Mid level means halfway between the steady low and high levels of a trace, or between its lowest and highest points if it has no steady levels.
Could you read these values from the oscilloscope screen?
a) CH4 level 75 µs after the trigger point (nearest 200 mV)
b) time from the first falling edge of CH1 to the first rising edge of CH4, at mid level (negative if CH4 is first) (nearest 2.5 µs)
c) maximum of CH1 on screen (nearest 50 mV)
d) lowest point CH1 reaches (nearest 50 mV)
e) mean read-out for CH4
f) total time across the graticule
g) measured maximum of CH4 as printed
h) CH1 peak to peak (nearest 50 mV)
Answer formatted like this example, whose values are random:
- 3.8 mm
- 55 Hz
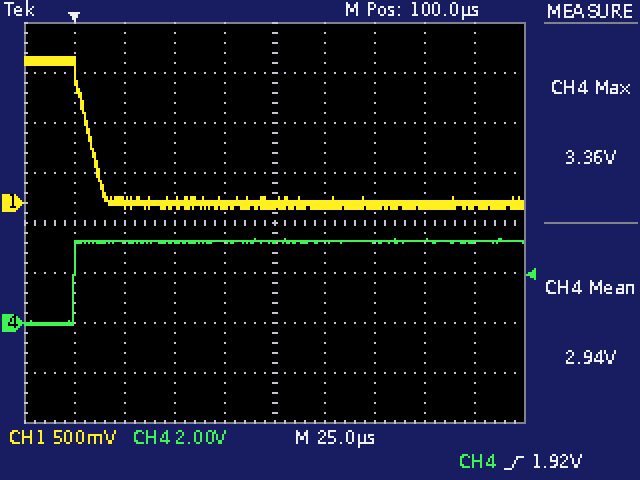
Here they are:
- 3.2 V
- -7.5 µs
- 1.45 V
- -50 mV
- 2.94 V
- 250 µs
- 3.36 V
- 1.50 V
